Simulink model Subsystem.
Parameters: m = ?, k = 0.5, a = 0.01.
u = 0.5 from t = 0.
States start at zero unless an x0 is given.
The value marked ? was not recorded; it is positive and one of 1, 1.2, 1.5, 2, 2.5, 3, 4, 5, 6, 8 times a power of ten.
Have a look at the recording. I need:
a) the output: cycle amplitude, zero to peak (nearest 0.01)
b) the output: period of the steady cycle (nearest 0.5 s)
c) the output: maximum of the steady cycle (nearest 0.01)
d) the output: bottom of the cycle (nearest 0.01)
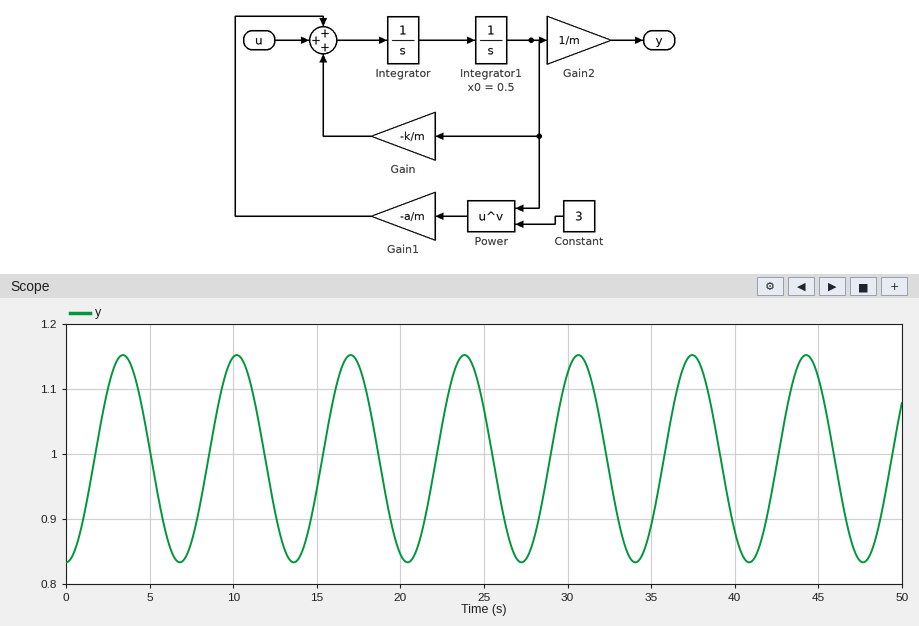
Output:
0.16
7.0 s
1.15
0.83
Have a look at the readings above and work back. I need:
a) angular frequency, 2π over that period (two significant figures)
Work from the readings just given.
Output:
0.90 rad/s
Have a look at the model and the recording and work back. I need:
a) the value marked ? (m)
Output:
0.6
